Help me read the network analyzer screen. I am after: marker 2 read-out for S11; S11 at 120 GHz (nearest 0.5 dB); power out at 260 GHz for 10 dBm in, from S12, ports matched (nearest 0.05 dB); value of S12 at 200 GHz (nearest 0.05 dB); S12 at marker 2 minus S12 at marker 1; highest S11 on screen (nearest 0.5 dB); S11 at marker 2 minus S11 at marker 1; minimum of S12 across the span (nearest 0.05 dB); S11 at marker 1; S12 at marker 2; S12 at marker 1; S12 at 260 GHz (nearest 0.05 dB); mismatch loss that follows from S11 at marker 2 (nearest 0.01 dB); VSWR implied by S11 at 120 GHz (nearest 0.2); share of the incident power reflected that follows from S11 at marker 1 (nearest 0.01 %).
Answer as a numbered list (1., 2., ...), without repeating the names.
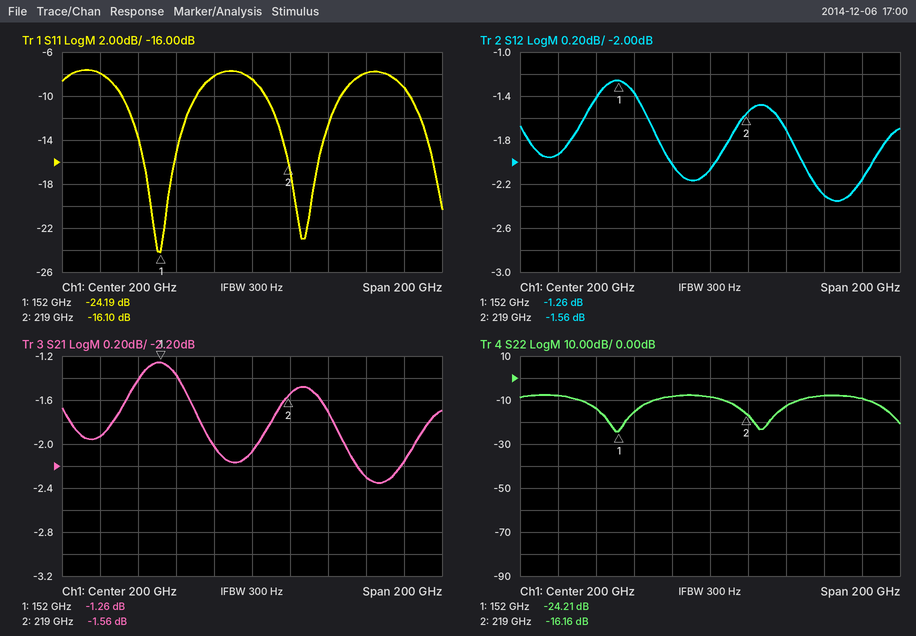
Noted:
1. -16.10 dB
2. -8.0 dB
3. 7.70 dBm
4. -2.05 dB
5. -0.30 dB
6. -7.5 dB
7. 8.09 dB
8. -2.35 dB
9. -24.19 dB
10. -1.56 dB
11. -1.26 dB
12. -2.30 dB
13. 0.11 dB
14. 2.4
15. 0.38 %
